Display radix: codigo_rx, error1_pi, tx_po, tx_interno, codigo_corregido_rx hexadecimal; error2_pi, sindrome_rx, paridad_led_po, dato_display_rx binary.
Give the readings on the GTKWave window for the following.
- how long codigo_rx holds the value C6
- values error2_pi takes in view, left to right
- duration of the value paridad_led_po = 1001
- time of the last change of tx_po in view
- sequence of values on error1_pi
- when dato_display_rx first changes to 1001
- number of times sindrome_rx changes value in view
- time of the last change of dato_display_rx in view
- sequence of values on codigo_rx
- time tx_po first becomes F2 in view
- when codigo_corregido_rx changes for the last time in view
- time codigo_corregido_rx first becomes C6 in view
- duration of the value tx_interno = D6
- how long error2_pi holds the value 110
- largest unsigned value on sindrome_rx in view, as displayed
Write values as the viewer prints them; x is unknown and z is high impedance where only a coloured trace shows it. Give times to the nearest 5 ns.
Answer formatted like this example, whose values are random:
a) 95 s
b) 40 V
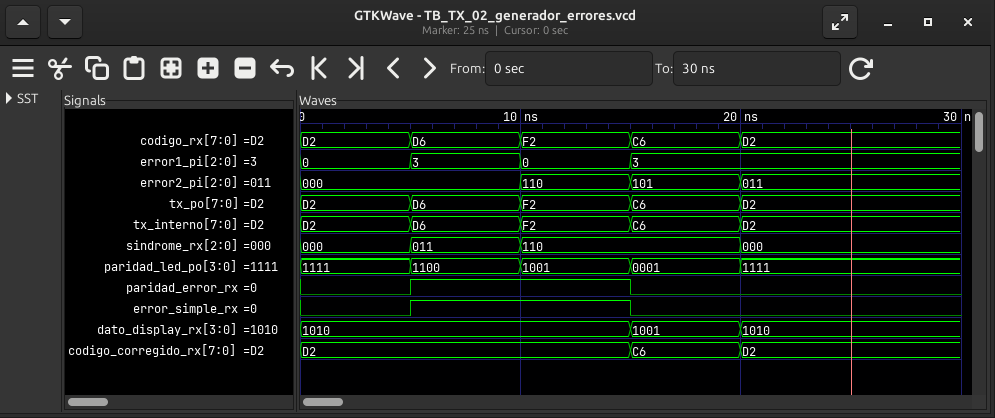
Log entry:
a) 5 ns
b) 000, 110, 101, 011
c) 5 ns
d) 20 ns
e) 0, 3, 0, 3
f) 15 ns
g) 3
h) 20 ns
i) D2, D6, F2, C6, D2
j) 10 ns
k) 20 ns
l) 15 ns
m) 5 ns
n) 5 ns
o) 110
